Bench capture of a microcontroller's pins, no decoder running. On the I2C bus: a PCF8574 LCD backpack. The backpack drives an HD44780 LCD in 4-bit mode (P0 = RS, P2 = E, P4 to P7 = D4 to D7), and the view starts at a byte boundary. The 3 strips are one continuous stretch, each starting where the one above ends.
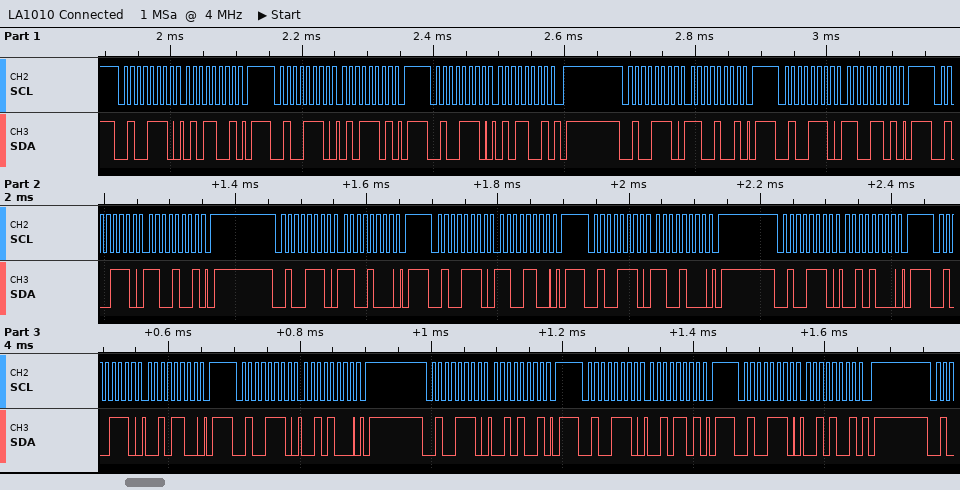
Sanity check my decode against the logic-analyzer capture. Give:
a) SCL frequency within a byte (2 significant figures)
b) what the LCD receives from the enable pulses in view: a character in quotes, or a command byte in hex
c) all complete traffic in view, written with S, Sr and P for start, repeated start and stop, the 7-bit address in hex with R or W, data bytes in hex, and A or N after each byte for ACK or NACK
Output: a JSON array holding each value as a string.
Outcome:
["100 kHz", "data 0x5C 0xC2", "S 27W A 59 A P S 27W A 5D A P S 27W A 59 A P S 27W A C9 A P S 27W A CD A P S 27W A C9 A P S 27W A C8 A P S 27W A CC A P S 27W A C8 A P S 27W A 28 A P S 27W A 2C A P S 27W A 28 A P S 27W A 29 A P S 27W A 2D A P S 27W A 29 A P"]
